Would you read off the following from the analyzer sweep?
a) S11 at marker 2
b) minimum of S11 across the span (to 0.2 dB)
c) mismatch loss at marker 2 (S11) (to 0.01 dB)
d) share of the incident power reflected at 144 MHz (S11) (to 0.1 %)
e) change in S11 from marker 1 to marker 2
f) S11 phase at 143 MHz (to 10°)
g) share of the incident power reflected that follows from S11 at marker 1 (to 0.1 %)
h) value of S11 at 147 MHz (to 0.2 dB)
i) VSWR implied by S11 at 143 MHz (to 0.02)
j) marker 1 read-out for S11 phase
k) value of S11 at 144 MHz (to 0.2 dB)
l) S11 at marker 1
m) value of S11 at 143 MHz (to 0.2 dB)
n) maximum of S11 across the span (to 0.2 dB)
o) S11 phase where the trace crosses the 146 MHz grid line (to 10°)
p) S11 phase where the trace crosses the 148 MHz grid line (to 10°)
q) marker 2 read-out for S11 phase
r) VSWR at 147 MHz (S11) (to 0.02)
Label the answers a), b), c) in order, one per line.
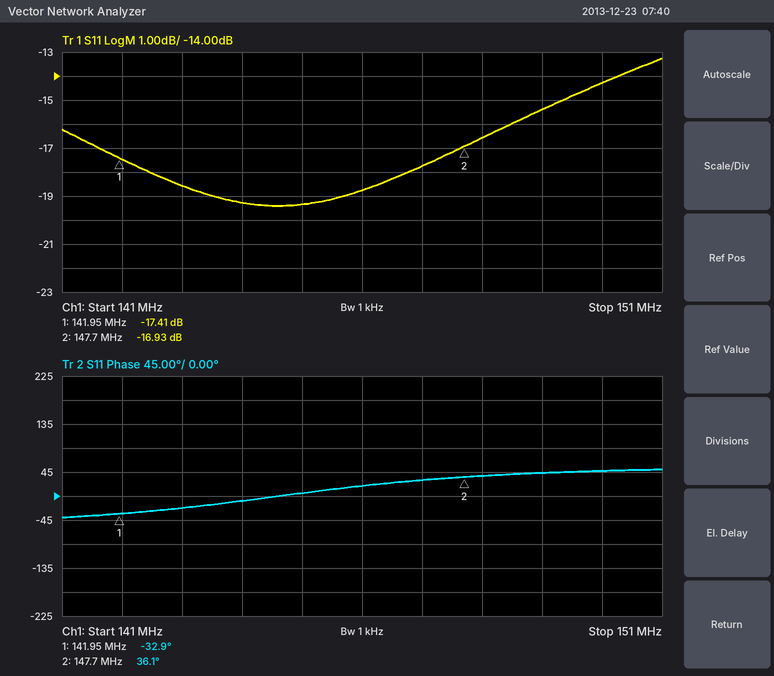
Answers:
a) -16.93 dB
b) -19.4 dB
c) 0.09 dB
d) 1.2 %
e) 0.48 dB
f) -20°
g) 1.8 %
h) -17.8 dB
i) 1.26
j) -32.9°
k) -19.2 dB
l) -17.41 dB
m) -18.6 dB
n) -13.2 dB
o) 20°
p) 40°
q) 36.1°
r) 1.30
